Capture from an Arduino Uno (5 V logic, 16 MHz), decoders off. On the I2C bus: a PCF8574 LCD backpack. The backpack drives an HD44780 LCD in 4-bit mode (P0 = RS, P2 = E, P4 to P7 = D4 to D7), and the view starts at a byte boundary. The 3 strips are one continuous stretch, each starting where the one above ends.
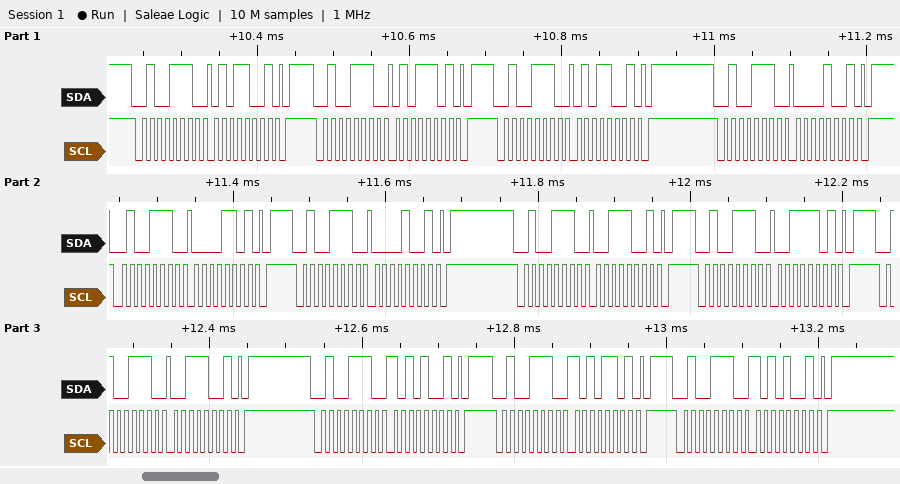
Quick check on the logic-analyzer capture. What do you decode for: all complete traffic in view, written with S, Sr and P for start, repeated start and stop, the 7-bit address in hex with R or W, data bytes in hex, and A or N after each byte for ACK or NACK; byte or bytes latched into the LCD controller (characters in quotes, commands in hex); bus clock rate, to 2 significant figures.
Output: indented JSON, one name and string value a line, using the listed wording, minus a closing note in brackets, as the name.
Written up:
{
  "all complete traffic in view, written with S, Sr and P for start, repeated start and stop, the 7-bit address in hex with R or W, data bytes in hex, and A or N after each byte for ACK or NACK": "S 27W A 59 A P S 27W A 5D A P S 27W A 59 A P S 27W A 09 A P S 27W A 0D A P S 27W A 09 A P S 27W A 39 A P S 27W A 3D A P S 27W A 39 A P S 27W A A9 A P S 27W A AD A P S 27W A A9 A P",
  "byte or bytes latched into the LCD controller": "'P' ':'",
  "bus clock rate, to 2 significant figures": "100 kHz"
}
